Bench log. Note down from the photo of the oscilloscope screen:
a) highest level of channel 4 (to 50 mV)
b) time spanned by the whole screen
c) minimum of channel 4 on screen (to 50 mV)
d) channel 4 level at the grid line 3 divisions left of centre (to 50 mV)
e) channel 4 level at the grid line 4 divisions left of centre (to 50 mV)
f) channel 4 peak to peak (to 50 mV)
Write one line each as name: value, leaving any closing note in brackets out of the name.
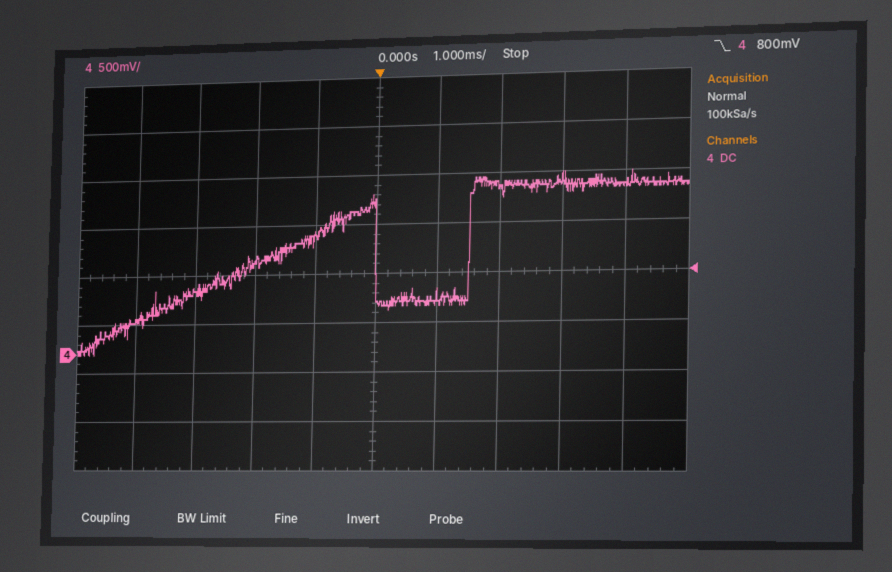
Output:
highest level of channel 4: 1.80 V
time spanned by the whole screen: 10 ms
minimum of channel 4 on screen: 0 mV
channel 4 level at the grid line 3 divisions left of centre: 650 mV
channel 4 level at the grid line 4 divisions left of centre: 350 mV
channel 4 peak to peak: 1.80 V
